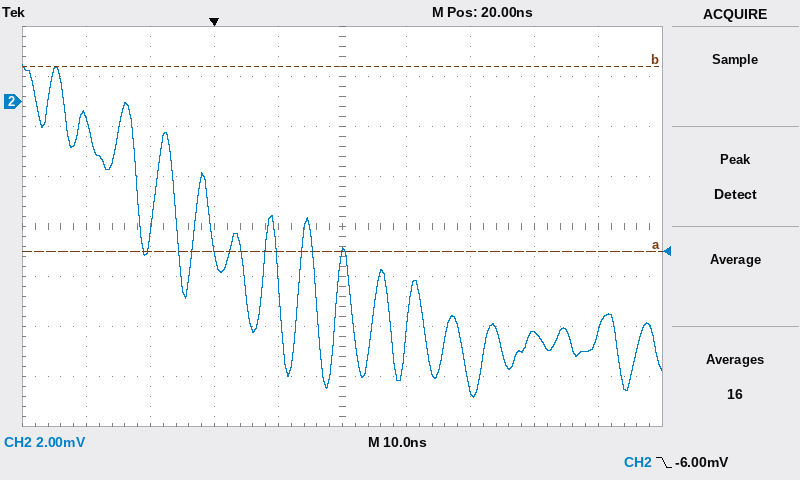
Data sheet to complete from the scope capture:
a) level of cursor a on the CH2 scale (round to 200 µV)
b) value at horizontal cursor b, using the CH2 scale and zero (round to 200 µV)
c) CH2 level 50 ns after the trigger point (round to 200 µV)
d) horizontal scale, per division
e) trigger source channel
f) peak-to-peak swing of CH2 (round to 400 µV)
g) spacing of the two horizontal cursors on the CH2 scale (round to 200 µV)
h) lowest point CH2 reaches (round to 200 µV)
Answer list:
-6.0 mV
1.4 mV
-9.2 mV
10 ns
CH2
13.2 mV
7.4 mV
-11.8 mV
